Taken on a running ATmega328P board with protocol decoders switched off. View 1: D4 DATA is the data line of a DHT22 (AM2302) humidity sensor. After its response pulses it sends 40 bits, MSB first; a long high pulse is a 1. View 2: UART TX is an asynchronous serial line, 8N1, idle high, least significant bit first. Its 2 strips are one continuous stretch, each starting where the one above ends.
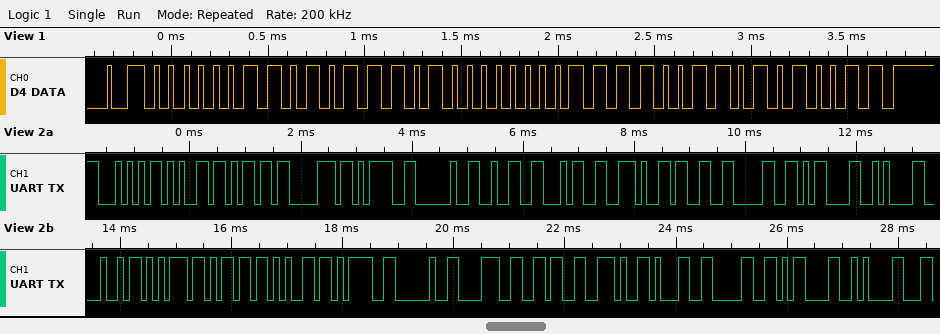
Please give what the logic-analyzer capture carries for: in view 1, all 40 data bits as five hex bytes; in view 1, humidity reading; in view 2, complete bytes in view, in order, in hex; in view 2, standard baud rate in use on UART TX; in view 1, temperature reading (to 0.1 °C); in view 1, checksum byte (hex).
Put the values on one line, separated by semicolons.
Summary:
03 5D 00 F3 53; 86.1 %; 54 65 6D 70 3D 20 32 34 2E 33 30 0D 0A 48 75 6D 65 3D 20 38 36 2E 31 30 0D 0A; 9600 baud; 24.3 °C; 0x53
